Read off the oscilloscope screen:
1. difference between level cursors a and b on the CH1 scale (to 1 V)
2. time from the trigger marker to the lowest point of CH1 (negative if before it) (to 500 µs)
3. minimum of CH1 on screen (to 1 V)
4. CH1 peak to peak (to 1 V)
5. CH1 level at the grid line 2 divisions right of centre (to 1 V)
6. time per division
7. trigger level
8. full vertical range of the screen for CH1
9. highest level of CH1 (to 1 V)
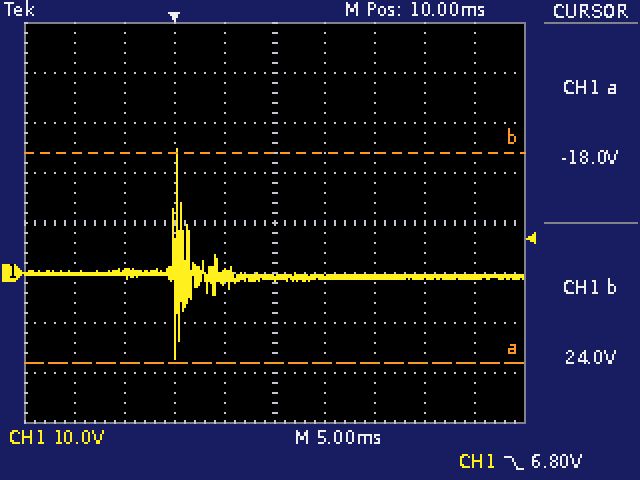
42 V
0.0 ms
-17 V
42 V
-1 V
5 ms
6.80 V
80 V
25 V
